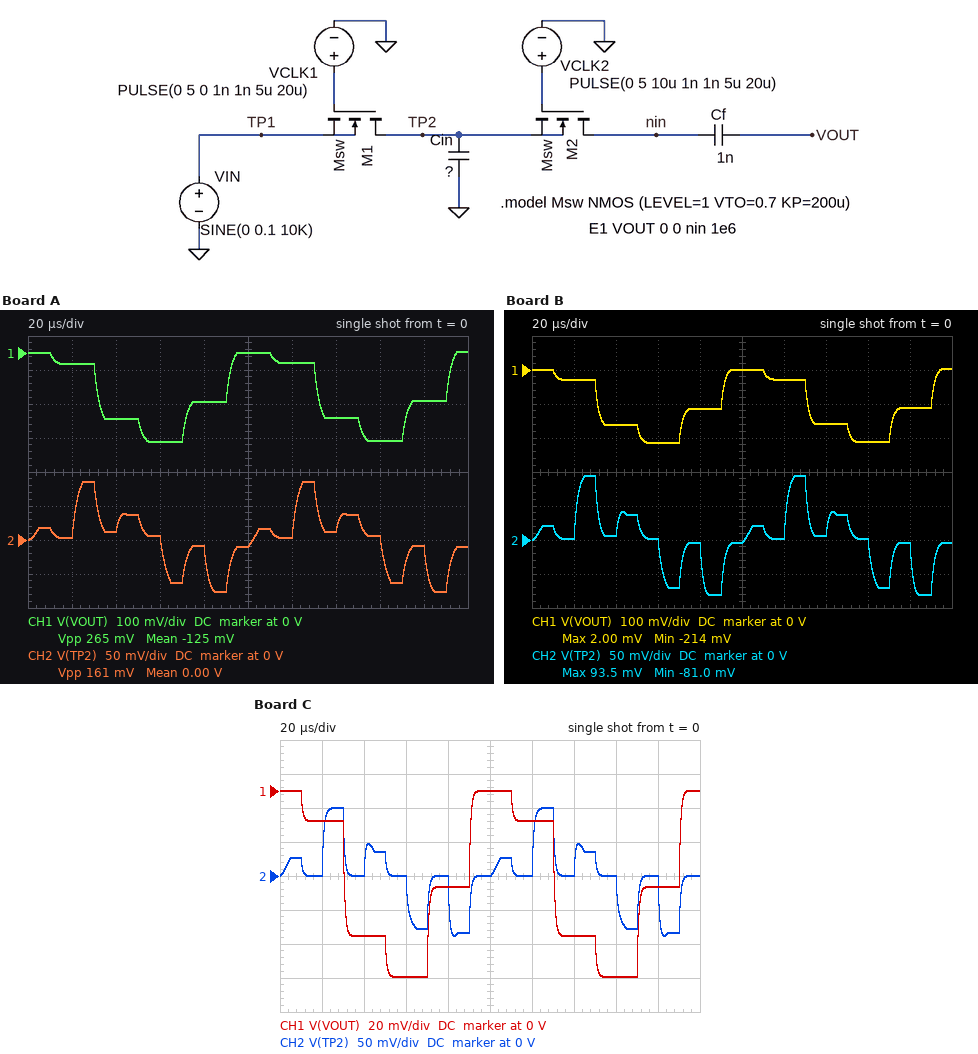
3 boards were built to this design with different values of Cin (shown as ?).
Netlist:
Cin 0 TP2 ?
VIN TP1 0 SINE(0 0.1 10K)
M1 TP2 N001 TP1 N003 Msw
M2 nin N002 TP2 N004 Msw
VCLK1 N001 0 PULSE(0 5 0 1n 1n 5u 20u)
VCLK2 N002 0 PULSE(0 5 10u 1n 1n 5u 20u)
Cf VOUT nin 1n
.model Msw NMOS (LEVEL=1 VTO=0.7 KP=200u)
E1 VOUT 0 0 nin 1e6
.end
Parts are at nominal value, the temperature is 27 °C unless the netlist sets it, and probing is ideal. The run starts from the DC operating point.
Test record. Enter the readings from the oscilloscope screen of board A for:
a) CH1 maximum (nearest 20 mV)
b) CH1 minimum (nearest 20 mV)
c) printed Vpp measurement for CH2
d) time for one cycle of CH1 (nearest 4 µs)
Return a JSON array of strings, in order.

["0 V", "-260 mV", "161 mV", "100 µs"]
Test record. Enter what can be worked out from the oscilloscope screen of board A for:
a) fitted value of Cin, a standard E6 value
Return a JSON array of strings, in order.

["2.2 nF"]
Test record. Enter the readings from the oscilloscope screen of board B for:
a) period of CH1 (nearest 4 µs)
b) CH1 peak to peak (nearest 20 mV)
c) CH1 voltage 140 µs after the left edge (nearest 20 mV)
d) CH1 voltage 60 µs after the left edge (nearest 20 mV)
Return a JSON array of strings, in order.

["100 µs", "220 mV", "-160 mV", "-220 mV"]
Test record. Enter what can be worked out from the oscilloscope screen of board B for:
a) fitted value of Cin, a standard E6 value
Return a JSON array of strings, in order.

["1.5 nF"]
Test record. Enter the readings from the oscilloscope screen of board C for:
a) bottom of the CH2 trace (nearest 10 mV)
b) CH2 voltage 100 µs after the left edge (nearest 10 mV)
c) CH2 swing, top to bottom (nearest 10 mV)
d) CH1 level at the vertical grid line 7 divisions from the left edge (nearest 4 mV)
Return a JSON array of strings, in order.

["-90 mV", "0 V", "190 mV", "-84 mV"]
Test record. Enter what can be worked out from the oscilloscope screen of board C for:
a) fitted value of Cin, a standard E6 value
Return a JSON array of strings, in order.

["680 pF"]
